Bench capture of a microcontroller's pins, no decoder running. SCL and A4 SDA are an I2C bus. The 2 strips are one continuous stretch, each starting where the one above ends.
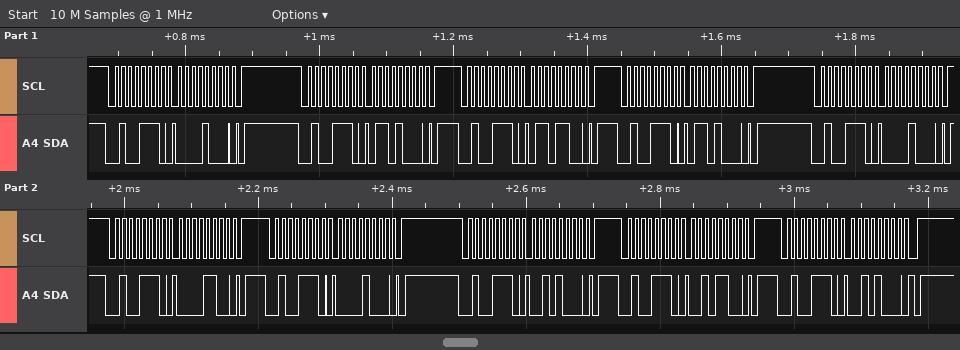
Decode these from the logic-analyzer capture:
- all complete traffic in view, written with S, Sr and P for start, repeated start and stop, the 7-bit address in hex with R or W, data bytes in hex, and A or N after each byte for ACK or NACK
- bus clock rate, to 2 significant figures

S 27W A 08 A P S 27W A 68 A P S 27W A 6C A P S 27W A 68 A P S 27W A 08 A P S 27W A 0C A P S 27W A 08 A P S 27W A 28 A P S 27W A 2C A P S 27W A 28 A P
100 kHz
